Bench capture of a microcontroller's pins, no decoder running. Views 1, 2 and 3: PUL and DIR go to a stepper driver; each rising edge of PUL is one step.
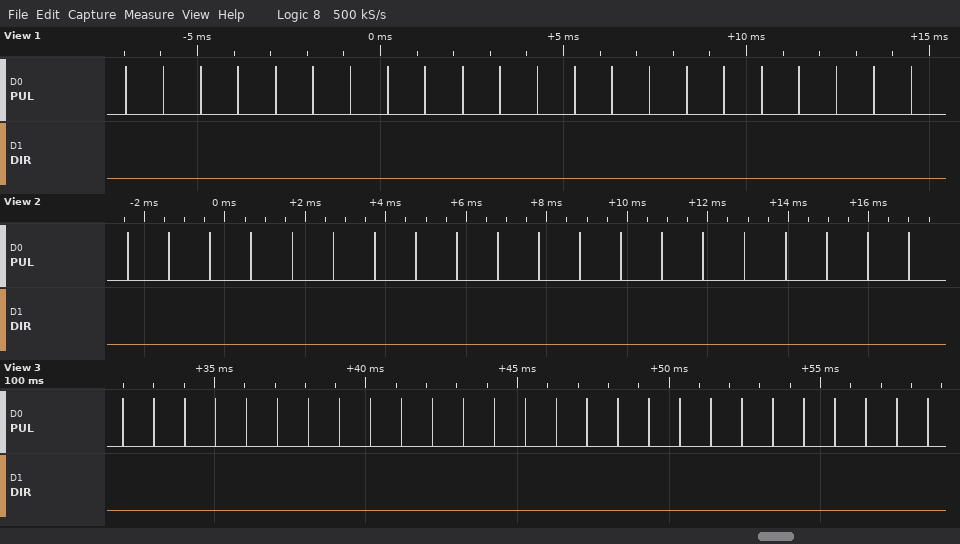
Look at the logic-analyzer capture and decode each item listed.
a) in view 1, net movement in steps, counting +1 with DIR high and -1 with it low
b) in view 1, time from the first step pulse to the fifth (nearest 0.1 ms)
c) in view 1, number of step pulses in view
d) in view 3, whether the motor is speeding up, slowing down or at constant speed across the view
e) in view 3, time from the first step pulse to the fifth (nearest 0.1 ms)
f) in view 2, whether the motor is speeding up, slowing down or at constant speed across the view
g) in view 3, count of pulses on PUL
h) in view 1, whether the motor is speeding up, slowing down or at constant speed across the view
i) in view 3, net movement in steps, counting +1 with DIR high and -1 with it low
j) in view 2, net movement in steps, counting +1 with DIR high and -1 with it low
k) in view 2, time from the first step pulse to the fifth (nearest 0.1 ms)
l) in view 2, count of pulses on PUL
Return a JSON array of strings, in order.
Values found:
["-22", "4.1 ms", "22", "constant speed", "4.1 ms", "constant speed", "27", "constant speed", "-27", "-20", "4.1 ms", "20"]
